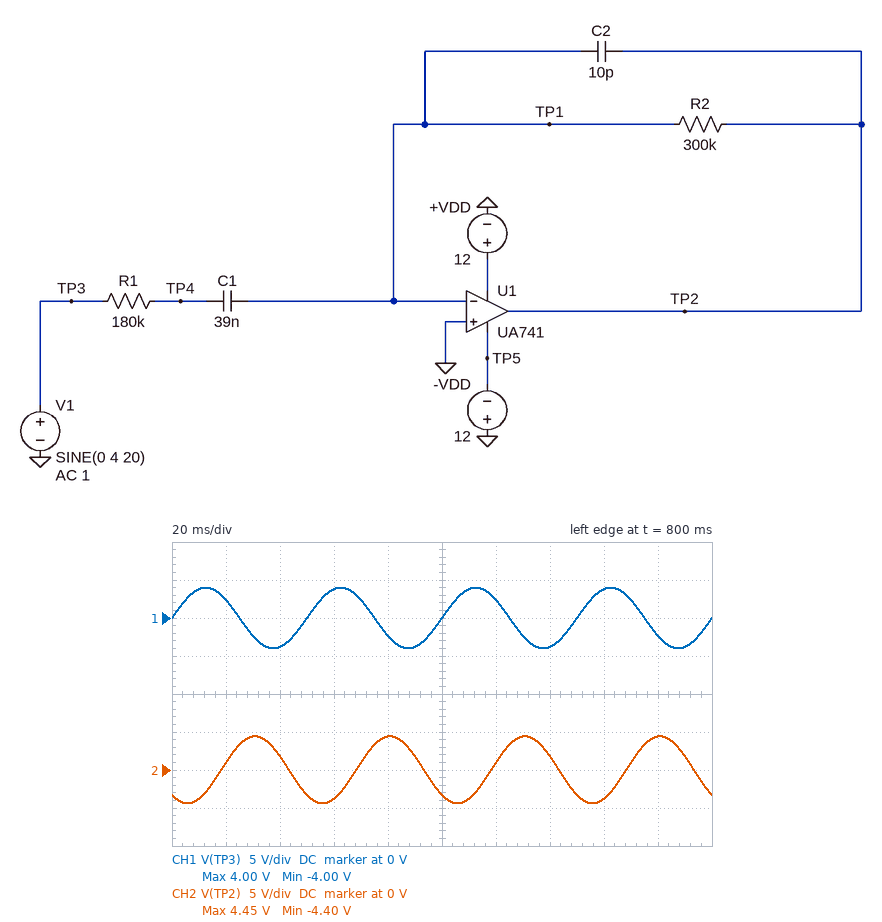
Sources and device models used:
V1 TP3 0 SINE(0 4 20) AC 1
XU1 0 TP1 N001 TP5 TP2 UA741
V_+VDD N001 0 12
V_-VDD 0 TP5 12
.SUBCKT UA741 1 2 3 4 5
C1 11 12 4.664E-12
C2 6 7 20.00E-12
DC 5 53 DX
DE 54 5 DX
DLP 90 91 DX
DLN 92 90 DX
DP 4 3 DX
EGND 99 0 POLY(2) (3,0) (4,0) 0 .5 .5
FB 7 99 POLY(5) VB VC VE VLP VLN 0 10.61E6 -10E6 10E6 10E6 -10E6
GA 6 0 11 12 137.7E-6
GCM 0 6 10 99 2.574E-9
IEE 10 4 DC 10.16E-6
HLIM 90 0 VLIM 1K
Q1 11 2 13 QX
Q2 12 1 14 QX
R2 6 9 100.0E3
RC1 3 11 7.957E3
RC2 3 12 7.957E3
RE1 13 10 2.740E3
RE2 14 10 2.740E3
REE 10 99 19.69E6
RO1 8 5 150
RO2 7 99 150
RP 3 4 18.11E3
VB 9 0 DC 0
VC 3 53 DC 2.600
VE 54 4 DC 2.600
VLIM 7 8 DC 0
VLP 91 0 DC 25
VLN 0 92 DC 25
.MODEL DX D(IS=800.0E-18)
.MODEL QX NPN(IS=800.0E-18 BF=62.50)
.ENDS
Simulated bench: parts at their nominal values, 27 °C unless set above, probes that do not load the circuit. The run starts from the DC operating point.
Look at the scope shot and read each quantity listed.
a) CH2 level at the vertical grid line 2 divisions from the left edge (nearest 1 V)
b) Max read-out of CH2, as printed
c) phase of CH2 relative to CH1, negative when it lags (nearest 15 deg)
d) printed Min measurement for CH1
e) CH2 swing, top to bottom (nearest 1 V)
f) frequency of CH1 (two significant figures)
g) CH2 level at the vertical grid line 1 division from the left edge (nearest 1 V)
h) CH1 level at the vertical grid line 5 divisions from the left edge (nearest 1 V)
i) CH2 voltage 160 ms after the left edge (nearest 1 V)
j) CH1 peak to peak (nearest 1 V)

2 V
4.45 V
-135 deg
-4.00 V
9 V
20 Hz
1 V
0 V
-4 V
8 V
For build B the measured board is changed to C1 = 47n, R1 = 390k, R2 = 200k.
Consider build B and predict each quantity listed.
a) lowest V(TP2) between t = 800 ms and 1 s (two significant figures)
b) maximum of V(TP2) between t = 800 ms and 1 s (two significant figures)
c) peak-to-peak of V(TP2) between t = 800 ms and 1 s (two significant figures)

-1.9 V
1.9 V
3.8 V
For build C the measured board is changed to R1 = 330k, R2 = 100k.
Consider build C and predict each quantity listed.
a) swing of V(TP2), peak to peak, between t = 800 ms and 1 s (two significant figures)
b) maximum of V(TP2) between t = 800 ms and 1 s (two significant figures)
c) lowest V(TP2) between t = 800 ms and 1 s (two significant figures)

2.1 V
1.0 V
-1.0 V
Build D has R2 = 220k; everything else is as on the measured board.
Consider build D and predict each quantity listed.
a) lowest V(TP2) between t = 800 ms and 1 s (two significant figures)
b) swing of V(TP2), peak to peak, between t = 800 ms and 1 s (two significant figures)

-3.2 V
6.5 V
